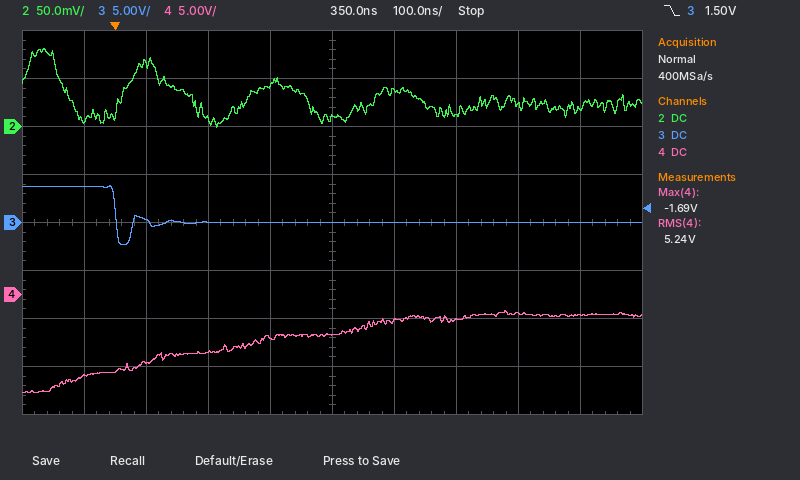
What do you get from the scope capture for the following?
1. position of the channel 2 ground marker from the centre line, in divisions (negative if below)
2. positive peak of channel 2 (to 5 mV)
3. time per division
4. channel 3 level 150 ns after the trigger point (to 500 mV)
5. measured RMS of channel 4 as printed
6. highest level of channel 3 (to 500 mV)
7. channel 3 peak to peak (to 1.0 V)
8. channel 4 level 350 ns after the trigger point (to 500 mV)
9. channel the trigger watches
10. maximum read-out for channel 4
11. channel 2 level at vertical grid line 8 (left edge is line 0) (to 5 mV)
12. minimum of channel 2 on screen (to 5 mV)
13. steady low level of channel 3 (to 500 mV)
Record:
+2.0 div
80 mV
100 ns
0.0 V
5.24 V
4.0 V
6.0 V
-4.0 V
channel 3
-1.69 V
20 mV
0 mV
0.0 V
